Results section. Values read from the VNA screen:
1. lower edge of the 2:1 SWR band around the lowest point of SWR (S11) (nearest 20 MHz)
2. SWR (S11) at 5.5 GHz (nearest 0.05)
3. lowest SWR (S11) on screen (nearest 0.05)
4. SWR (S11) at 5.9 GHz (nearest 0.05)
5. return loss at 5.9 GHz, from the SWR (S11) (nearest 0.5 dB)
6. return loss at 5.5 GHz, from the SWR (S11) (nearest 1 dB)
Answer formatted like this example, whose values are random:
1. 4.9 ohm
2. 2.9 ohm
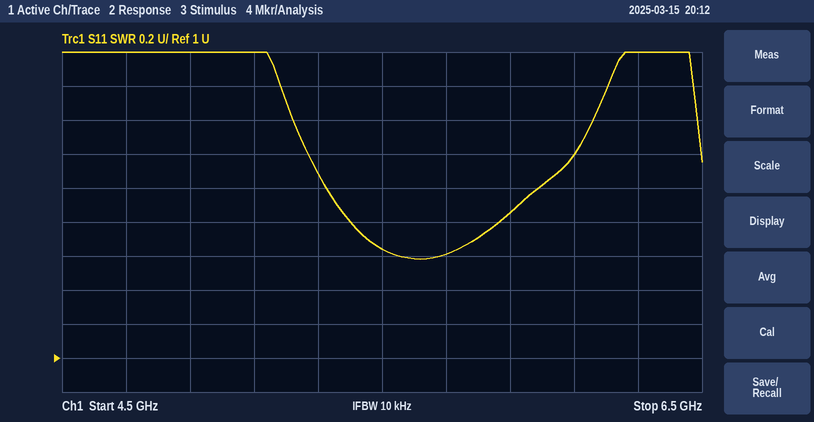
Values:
1. 5.32 GHz
2. 1.65
3. 1.60
4. 1.85
5. 10.5 dB
6. 12 dB
